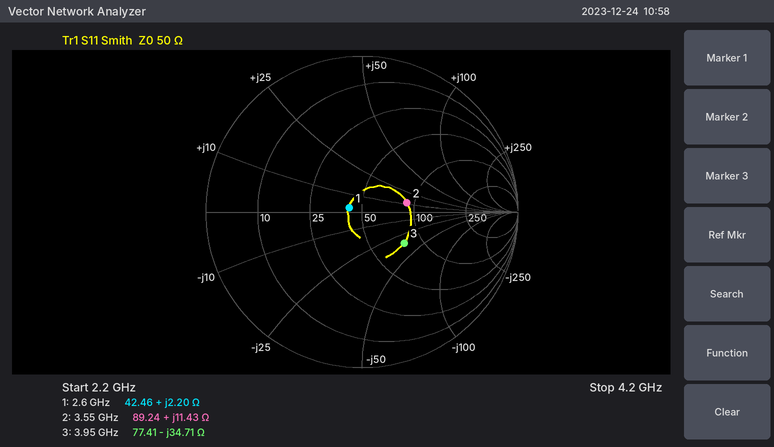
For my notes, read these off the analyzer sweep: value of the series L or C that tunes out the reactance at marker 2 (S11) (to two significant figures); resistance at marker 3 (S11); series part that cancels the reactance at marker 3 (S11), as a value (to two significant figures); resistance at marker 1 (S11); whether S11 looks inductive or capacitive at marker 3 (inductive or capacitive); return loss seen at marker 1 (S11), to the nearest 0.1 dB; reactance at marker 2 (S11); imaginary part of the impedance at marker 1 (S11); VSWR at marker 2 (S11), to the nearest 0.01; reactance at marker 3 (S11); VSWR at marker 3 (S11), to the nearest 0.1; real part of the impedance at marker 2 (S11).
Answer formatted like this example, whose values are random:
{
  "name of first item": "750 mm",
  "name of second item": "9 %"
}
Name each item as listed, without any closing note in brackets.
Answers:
{
  "value of the series L or C that tunes out the reactance at marker 2 (S11)": "3.9 pF",
  "resistance at marker 3": "77.41 Ω",
  "series part that cancels the reactance at marker 3 (S11), as a value": "1.4 nH",
  "resistance at marker 1": "42.46 Ω",
  "whether S11 looks inductive or capacitive at marker 3": "capacitive",
  "return loss seen at marker 1 (S11), to the nearest 0.1 dB": "21.4 dB",
  "reactance at marker 2": "+11.43 Ω",
  "imaginary part of the impedance at marker 1": "+2.20 Ω",
  "VSWR at marker 2 (S11), to the nearest 0.01": "1.83",
  "reactance at marker 3": "-34.71 Ω",
  "VSWR at marker 3 (S11), to the nearest 0.1": "2.0",
  "real part of the impedance at marker 2": "89.24 Ω"
}
